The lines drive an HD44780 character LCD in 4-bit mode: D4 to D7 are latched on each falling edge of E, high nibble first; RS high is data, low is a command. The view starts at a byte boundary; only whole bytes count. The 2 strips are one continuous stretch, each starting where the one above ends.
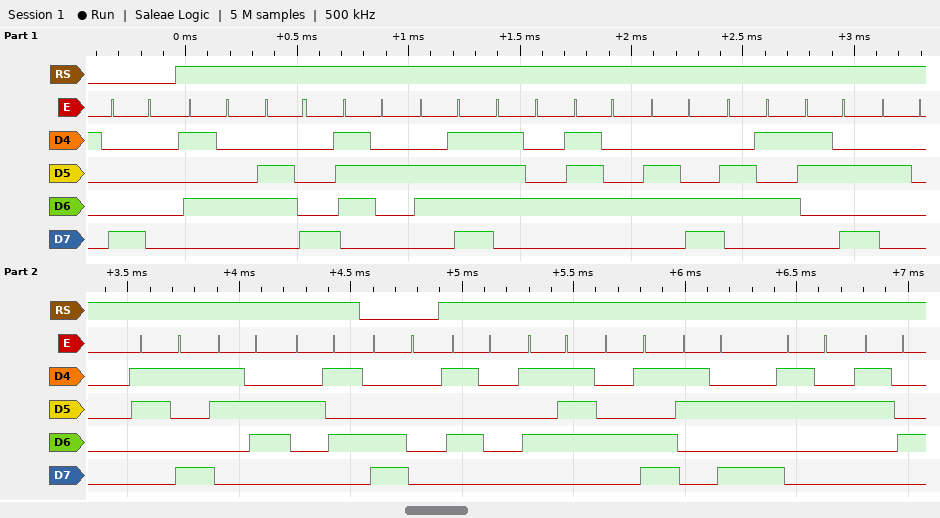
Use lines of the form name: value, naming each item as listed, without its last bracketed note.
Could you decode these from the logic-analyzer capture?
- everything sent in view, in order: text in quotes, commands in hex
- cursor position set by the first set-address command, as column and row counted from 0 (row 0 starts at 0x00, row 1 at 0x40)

everything sent in view, in order: text in quotes, commands in hex: 0x80 "Throttle: 96%" 0xC0 "PWM:24"
cursor position set by the first set-address command, as column and row counted from 0: column 0, row 0
